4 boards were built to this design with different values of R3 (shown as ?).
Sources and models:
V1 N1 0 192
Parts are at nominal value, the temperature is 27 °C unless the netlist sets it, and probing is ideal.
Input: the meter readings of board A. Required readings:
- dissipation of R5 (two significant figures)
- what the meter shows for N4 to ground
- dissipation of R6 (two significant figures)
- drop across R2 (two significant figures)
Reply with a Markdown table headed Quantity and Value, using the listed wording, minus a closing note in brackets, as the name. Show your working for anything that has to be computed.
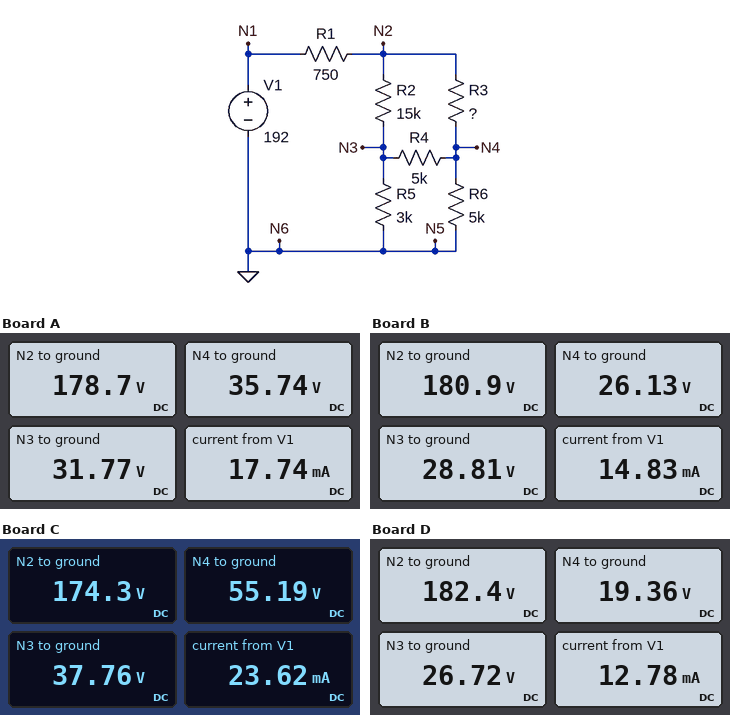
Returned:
| Quantity | Value |
|---|---|
| dissipation of R5 | (31.77 V)^2 / 3 kΩ = 340 mW |
| what the meter shows for N4 to ground | 35.74 V |
| dissipation of R6 | (35.74 V)^2 / 5 kΩ = 260 mW |
| drop across R2 | 178.7 V - 31.77 V = 150 V |
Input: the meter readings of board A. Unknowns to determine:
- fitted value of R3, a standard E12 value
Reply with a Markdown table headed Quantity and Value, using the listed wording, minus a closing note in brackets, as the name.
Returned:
| Quantity | Value |
|---|---|
| fitted value of R3, a standard E12 value | 18 kΩ |
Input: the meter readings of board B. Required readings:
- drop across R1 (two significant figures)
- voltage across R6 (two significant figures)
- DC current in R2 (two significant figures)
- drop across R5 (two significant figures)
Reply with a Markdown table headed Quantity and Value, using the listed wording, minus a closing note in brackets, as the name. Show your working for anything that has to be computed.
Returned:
| Quantity | Value |
|---|---|
| drop across R1 | 192 V - 180.9 V = 11 V |
| voltage across R6 | 26.13 V = 26 V |
| DC current in R2 | (180.9 V - 28.81 V) / 15 kΩ = 10 mA |
| drop across R5 | 28.81 V = 29 V |
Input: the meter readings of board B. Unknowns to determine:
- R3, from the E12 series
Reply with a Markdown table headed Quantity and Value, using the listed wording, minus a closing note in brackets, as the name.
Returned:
| Quantity | Value |
|---|---|
| R3, from the E12 series | 33 kΩ |
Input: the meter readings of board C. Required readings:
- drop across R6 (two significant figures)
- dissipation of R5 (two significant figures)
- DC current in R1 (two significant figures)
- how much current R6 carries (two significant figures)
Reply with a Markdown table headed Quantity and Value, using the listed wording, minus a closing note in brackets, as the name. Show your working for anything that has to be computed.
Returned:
| Quantity | Value |
|---|---|
| drop across R6 | 55.19 V = 55 V |
| dissipation of R5 | (37.76 V)^2 / 3 kΩ = 480 mW |
| DC current in R1 | (192 V - 174.3 V) / 750 Ω = 24 mA |
| how much current R6 carries | (55.19 V) / 5 kΩ = 11 mA |
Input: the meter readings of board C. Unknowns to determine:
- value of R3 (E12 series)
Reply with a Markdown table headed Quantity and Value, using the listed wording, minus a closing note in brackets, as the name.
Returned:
| Quantity | Value |
|---|---|
| value of R3 | 8.2 kΩ |
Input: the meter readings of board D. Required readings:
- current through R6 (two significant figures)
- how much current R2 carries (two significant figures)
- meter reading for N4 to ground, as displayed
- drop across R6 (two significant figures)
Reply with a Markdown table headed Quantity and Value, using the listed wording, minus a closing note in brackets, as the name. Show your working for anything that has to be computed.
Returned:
| Quantity | Value |
|---|---|
| current through R6 | (19.36 V) / 5 kΩ = 3.9 mA |
| how much current R2 carries | (182.4 V - 26.72 V) / 15 kΩ = 10 mA |
| meter reading for N4 to ground, as displayed | 19.36 V |
| drop across R6 | 19.36 V = 19 V |
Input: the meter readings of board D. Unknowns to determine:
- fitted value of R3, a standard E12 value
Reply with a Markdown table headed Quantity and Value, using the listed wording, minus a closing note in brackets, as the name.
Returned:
| Quantity | Value |
|---|---|
| fitted value of R3, a standard E12 value | 68 kΩ |
